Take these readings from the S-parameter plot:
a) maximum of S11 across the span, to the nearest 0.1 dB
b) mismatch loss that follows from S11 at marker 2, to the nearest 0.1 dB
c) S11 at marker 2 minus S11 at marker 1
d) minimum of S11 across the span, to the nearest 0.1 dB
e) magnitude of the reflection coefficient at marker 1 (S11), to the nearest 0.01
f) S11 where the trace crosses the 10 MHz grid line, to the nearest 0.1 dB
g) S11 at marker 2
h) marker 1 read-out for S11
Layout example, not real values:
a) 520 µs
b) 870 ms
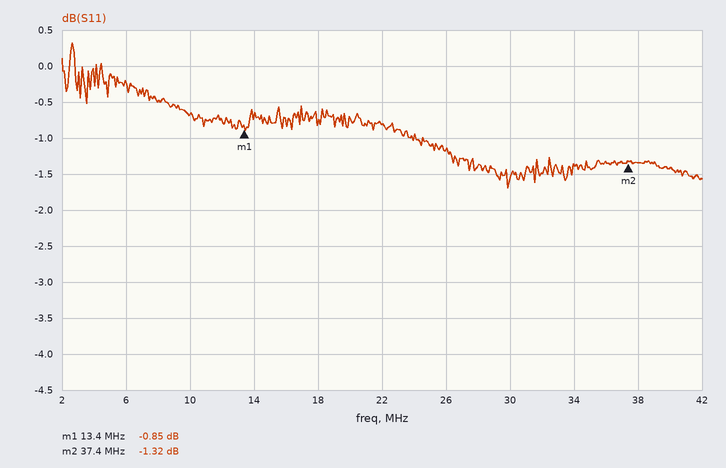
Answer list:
a) 0.3 dB
b) 5.8 dB
c) -0.47 dB
d) -1.7 dB
e) 0.91
f) -0.7 dB
g) -1.32 dB
h) -0.85 dB
